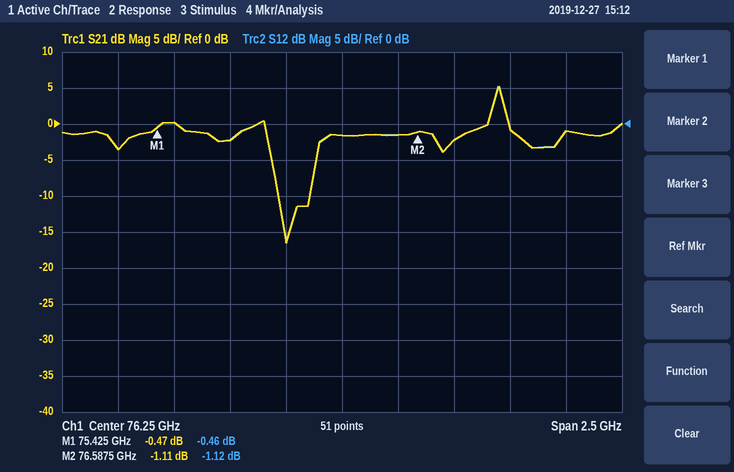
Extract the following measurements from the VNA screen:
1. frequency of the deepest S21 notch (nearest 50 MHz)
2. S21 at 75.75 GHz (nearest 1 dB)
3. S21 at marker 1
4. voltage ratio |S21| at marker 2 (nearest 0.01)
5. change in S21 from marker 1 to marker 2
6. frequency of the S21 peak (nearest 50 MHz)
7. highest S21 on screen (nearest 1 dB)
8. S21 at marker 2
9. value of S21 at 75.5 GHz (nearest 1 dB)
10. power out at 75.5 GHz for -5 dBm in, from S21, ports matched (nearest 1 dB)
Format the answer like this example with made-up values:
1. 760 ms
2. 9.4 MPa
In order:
1. 76.00 GHz
2. -2 dB
3. -0.47 dB
4. 0.88
5. -0.64 dB
6. 76.95 GHz
7. 5 dB
8. -1.11 dB
9. 0 dB
10. -5 dBm
